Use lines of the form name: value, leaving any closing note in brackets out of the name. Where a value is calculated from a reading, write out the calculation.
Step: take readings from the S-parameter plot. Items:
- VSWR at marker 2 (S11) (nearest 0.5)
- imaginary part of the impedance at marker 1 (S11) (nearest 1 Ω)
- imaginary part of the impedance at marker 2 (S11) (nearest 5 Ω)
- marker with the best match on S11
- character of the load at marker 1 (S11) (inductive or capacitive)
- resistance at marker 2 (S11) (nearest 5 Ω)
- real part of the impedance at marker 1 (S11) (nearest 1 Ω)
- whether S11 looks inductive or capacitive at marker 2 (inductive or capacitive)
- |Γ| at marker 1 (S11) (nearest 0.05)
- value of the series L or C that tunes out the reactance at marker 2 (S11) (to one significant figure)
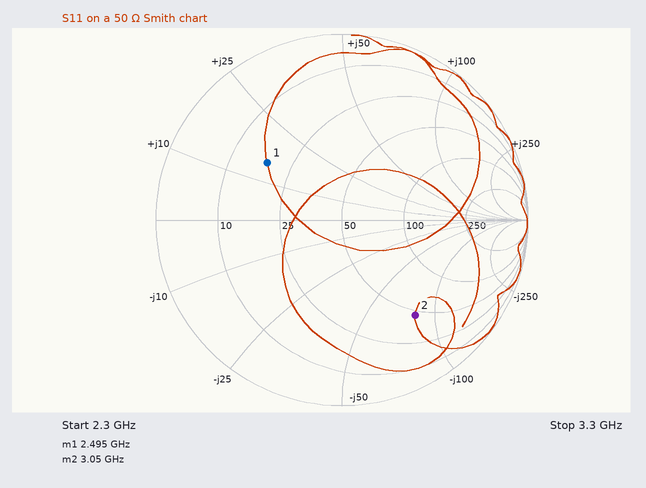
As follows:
VSWR at marker 2 (S11): 4.5
imaginary part of the impedance at marker 1 (S11): +15 Ω
imaginary part of the impedance at marker 2 (S11): -80 Ω
marker with the best match on S11: marker 1
character of the load at marker 1 (S11): inductive
resistance at marker 2 (S11): 45 Ω
real part of the impedance at marker 1 (S11): 18 Ω
whether S11 looks inductive or capacitive at marker 2: capacitive
|Γ| at marker 1 (S11): 0.50
value of the series L or C that tunes out the reactance at marker 2 (S11): L = 80 Ω/(2π × 3.05 GHz) ≈ 4 nH
